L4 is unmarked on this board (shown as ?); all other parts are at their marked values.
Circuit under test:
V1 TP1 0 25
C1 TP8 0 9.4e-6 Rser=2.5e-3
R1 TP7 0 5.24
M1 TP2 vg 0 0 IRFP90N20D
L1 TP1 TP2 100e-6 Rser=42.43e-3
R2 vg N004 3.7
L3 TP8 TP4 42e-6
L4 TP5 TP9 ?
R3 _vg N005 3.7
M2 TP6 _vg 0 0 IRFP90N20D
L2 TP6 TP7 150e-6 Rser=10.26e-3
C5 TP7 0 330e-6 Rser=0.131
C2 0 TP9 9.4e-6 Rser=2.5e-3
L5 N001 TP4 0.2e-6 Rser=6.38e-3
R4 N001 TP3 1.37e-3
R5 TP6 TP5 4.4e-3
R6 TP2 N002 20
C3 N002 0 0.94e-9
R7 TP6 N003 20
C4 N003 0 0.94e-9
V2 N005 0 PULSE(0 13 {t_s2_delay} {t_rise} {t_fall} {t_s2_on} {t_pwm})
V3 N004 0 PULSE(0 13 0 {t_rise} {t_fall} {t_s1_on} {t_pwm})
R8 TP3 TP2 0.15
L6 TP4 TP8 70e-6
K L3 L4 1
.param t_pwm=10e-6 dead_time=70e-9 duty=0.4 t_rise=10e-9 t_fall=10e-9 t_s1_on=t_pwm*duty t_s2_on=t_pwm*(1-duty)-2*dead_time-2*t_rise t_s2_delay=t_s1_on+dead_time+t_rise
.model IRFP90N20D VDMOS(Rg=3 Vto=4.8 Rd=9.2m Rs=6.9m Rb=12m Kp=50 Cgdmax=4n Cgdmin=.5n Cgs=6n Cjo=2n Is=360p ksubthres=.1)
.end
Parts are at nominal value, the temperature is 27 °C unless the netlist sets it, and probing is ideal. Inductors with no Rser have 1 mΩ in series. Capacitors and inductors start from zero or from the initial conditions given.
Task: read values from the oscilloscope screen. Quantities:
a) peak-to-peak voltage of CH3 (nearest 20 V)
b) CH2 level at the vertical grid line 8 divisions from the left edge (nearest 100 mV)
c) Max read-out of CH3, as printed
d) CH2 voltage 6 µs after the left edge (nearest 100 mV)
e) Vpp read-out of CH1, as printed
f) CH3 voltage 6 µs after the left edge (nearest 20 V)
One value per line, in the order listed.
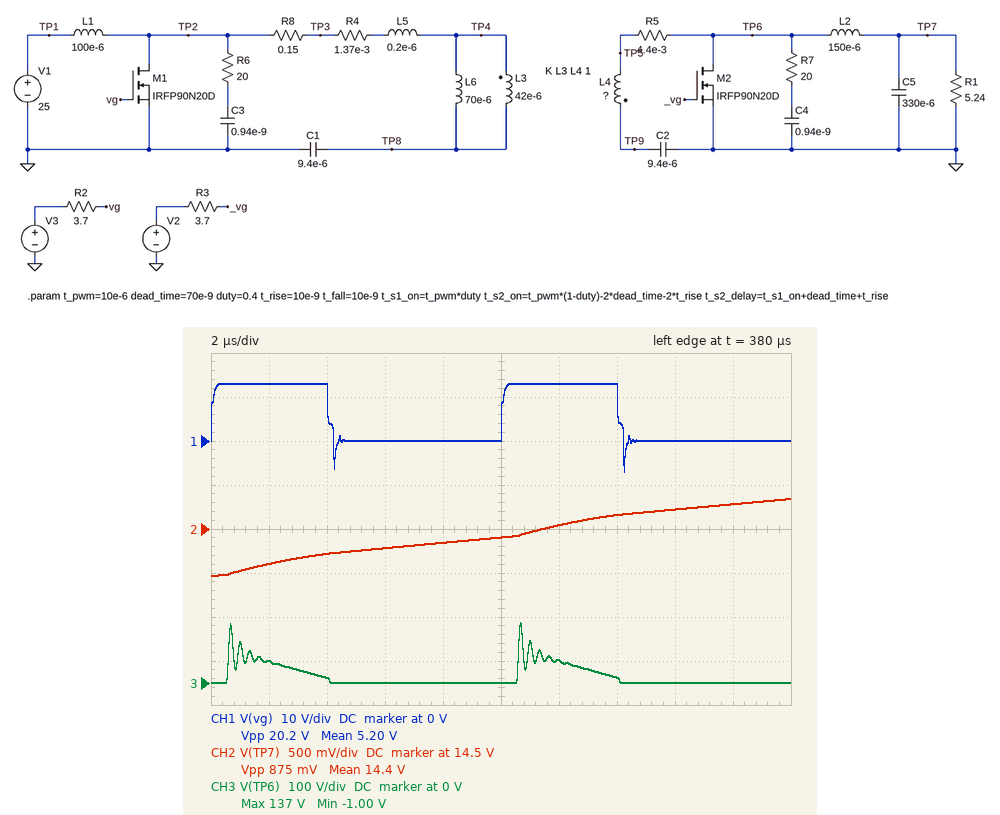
140 V
14.7 V
137 V
14.3 V
20.2 V
0 V
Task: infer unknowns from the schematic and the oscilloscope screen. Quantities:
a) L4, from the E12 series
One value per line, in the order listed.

330 µH
